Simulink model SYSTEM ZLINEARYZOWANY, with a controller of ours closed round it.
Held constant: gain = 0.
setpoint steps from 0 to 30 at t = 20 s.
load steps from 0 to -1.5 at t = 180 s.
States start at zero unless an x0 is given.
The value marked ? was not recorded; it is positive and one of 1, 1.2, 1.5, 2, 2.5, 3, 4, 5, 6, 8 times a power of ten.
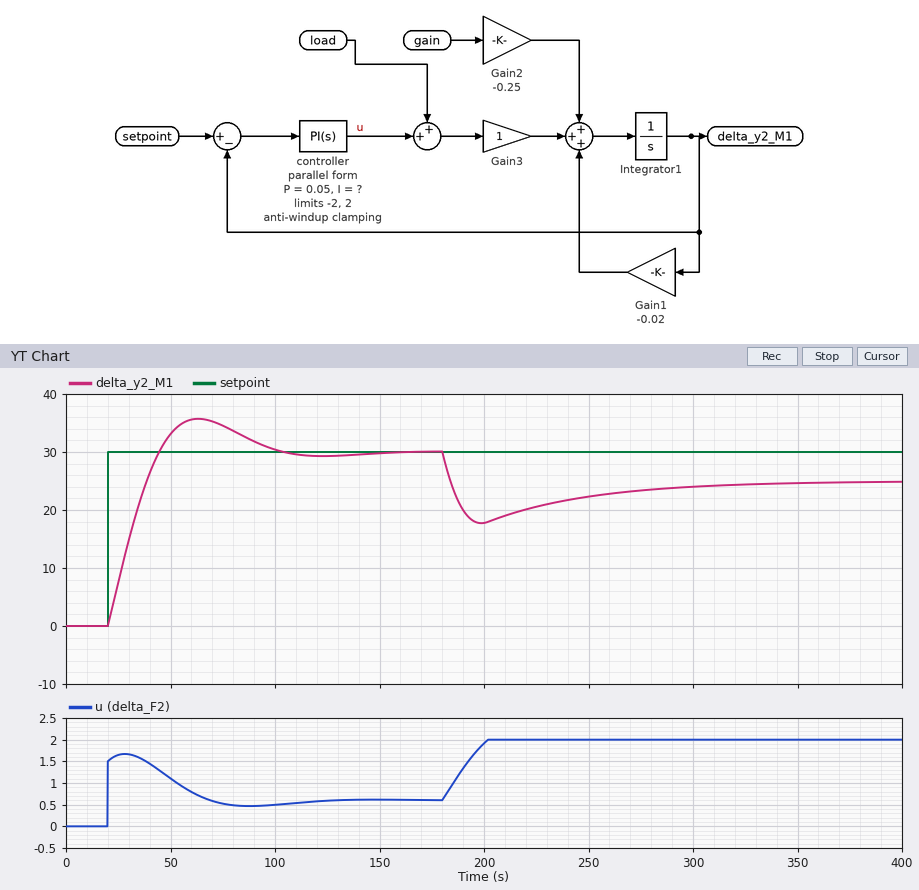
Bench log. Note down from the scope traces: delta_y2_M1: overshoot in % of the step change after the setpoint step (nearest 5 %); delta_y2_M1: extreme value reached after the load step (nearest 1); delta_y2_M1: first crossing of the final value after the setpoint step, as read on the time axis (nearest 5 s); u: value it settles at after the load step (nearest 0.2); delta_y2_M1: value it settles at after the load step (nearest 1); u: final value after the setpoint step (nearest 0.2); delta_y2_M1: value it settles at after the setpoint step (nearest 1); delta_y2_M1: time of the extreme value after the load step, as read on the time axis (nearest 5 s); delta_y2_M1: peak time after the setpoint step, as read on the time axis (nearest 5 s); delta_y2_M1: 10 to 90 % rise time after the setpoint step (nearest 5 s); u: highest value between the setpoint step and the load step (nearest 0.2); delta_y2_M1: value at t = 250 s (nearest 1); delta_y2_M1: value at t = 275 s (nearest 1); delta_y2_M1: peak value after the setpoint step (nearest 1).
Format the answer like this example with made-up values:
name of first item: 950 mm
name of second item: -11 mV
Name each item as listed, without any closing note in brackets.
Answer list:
delta_y2_M1: overshoot in % of the step change after the setpoint step: 20 %
delta_y2_M1: extreme value reached after the load step: 18
delta_y2_M1: first crossing of the final value after the setpoint step, as read on the time axis: 45 s
u: value it settles at after the load step: 2.0
delta_y2_M1: value it settles at after the load step: 25
u: final value after the setpoint step: 0.6
delta_y2_M1: value it settles at after the setpoint step: 30
delta_y2_M1: time of the extreme value after the load step, as read on the time axis: 200 s
delta_y2_M1: peak time after the setpoint step, as read on the time axis: 65 s
delta_y2_M1: 10 to 90 % rise time after the setpoint step: 20 s
u: highest value between the setpoint step and the load step: 1.6
delta_y2_M1: value at t = 250 s: 22
delta_y2_M1: value at t = 275 s: 23
delta_y2_M1: peak value after the setpoint step: 36
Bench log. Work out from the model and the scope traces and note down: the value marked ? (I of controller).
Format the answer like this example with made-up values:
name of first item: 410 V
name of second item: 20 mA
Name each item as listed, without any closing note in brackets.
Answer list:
the value marked ?: 0.004
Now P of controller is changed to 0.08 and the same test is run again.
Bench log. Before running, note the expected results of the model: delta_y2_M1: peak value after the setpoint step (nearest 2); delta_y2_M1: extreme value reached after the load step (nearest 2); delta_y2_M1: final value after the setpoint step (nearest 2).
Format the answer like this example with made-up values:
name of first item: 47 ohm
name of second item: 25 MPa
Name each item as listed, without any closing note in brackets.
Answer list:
delta_y2_M1: peak value after the setpoint step: 32
delta_y2_M1: extreme value reached after the load step: 20
delta_y2_M1: final value after the setpoint step: 30
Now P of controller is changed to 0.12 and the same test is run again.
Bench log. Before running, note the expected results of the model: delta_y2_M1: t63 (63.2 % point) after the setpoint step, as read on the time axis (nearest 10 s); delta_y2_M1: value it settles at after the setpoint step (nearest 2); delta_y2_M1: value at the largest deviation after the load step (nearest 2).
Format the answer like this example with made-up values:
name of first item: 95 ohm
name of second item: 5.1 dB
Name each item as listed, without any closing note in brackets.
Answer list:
delta_y2_M1: t63 (63.2 % point) after the setpoint step, as read on the time axis: 30 s
delta_y2_M1: value it settles at after the setpoint step: 30
delta_y2_M1: value at the largest deviation after the load step: 22
